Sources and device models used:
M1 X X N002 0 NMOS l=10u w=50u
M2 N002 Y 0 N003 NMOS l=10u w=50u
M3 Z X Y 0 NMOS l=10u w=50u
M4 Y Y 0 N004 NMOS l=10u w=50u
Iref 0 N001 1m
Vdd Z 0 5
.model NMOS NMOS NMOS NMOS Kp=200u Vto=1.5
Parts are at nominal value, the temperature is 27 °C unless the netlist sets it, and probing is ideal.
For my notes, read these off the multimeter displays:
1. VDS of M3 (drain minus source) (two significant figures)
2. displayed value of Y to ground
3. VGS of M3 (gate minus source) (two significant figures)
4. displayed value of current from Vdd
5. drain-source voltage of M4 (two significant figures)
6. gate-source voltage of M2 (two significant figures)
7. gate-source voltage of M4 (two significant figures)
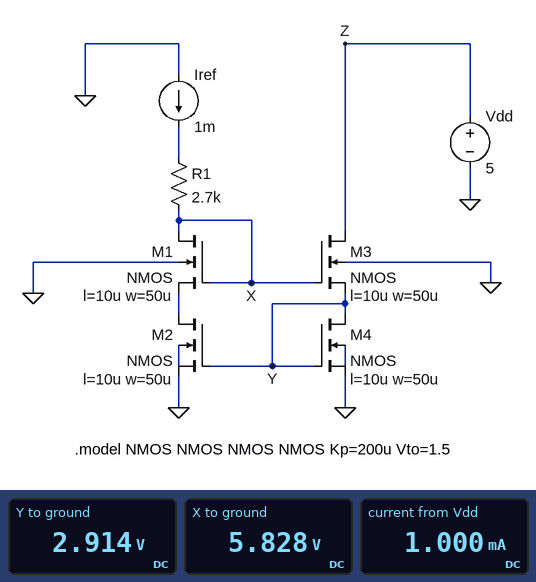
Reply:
2.1 V
2.914 V
2.9 V
1.000 mA
2.9 V
2.9 V
2.9 V
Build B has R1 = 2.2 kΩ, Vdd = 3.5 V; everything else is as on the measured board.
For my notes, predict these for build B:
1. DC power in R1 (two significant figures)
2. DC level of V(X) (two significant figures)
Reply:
2.2 mW
6.4 V
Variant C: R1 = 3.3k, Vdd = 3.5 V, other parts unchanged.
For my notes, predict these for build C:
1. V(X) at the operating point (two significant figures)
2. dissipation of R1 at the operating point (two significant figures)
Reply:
6.4 V
3.3 mW
